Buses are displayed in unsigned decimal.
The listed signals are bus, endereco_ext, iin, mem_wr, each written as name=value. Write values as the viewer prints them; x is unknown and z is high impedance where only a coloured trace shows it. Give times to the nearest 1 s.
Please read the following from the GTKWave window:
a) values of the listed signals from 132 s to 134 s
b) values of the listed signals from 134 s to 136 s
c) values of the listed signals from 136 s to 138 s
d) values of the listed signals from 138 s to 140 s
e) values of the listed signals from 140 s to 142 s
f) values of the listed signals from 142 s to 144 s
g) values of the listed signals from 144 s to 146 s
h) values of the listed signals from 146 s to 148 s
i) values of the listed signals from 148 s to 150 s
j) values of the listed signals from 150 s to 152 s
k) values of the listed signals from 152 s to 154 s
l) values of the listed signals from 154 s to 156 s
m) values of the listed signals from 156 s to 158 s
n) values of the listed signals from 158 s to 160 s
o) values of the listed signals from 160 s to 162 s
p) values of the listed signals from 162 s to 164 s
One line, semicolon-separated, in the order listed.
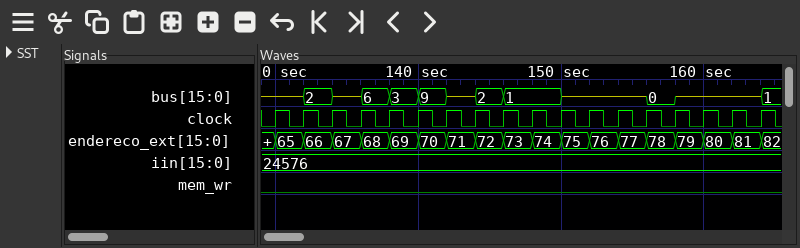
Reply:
bus=2, endereco_ext=66, iin=24576, mem_wr=0; bus=z, endereco_ext=67, iin=24576, mem_wr=0; bus=6, endereco_ext=68, iin=24576, mem_wr=0; bus=3, endereco_ext=69, iin=24576, mem_wr=0; bus=9, endereco_ext=70, iin=24576, mem_wr=0; bus=z, endereco_ext=71, iin=24576, mem_wr=0; bus=2, endereco_ext=72, iin=24576, mem_wr=0; bus=1, endereco_ext=73, iin=24576, mem_wr=0; bus=1, endereco_ext=74, iin=24576, mem_wr=0; bus=z, endereco_ext=75, iin=24576, mem_wr=0; bus=z, endereco_ext=76, iin=24576, mem_wr=0; bus=z, endereco_ext=77, iin=24576, mem_wr=0; bus=0, endereco_ext=78, iin=24576, mem_wr=0; bus=z, endereco_ext=79, iin=24576, mem_wr=0; bus=z, endereco_ext=80, iin=24576, mem_wr=0; bus=z, endereco_ext=81, iin=24576, mem_wr=0
